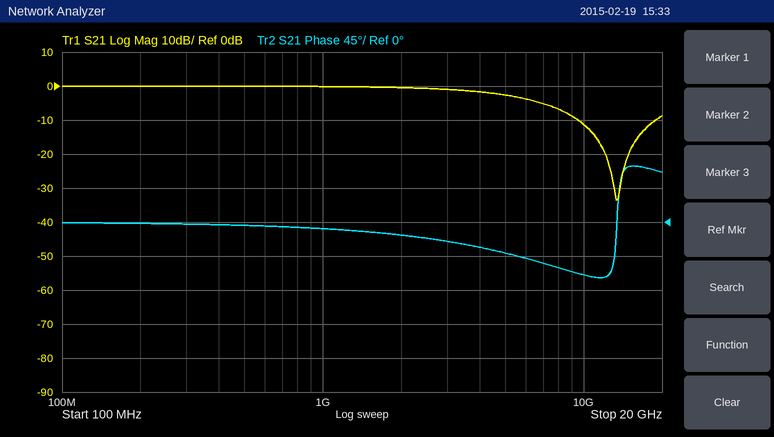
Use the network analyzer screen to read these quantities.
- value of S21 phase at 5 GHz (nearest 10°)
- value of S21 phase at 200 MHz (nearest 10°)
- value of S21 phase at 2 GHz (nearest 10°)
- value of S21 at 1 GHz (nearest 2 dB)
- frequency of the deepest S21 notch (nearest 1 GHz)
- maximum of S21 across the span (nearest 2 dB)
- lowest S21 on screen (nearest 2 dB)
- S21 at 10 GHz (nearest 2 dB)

-40°
0°
-20°
0 dB
13 GHz
0 dB
-34 dB
-12 dB
